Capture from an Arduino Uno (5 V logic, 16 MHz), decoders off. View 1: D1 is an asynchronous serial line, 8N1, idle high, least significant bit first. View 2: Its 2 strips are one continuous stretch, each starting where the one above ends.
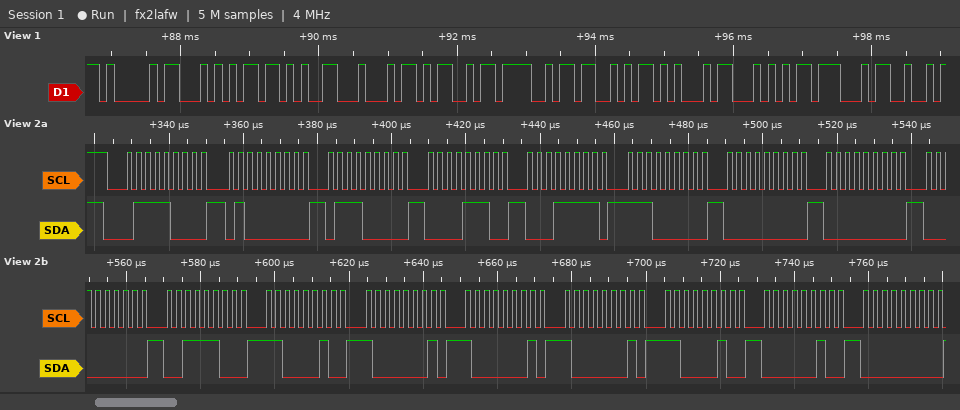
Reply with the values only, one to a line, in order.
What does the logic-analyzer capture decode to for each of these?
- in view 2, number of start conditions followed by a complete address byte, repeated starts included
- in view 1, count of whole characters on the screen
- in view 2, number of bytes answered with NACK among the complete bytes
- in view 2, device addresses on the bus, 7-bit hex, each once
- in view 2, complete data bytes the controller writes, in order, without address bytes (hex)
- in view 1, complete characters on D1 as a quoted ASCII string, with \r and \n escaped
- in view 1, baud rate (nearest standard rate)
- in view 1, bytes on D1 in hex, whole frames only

1
10
0
0x3C
40 70 0E 1F E0 00 00 00 3C C2 81 81 81 C2 02 00
"AT+DMOSETG"
9600 baud
0x41 0x54 0x2B 0x44 0x4D 0x4F 0x53 0x45 0x54 0x47
